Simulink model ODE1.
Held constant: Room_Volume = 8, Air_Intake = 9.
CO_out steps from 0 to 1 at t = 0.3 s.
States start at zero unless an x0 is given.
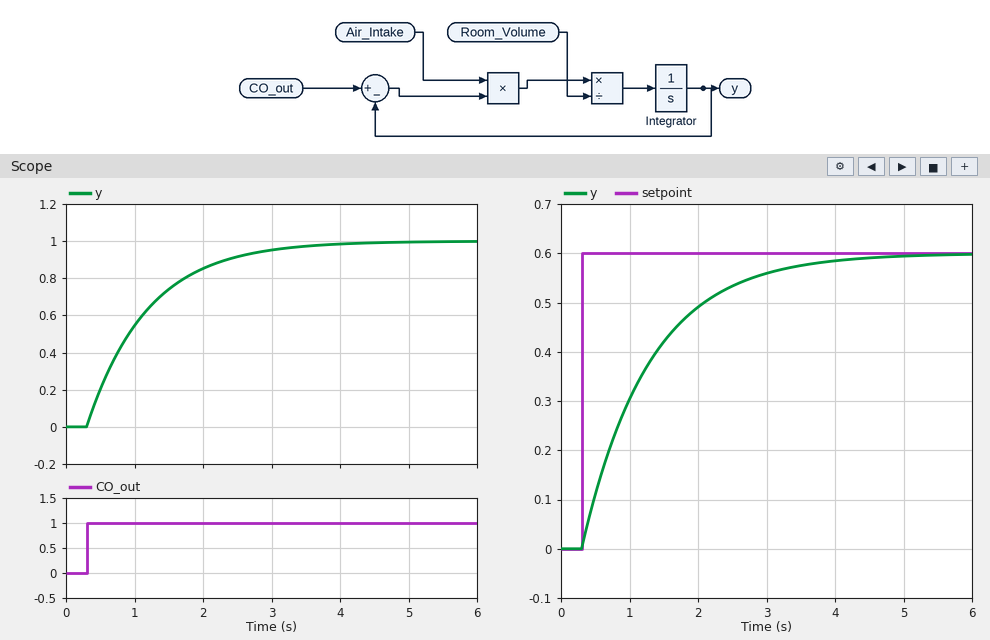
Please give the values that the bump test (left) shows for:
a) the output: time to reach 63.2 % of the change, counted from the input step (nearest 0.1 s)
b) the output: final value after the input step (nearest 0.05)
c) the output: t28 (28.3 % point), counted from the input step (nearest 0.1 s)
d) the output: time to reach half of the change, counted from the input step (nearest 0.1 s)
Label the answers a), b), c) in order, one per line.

a) 0.9 s
b) 1.00
c) 0.3 s
d) 0.6 s
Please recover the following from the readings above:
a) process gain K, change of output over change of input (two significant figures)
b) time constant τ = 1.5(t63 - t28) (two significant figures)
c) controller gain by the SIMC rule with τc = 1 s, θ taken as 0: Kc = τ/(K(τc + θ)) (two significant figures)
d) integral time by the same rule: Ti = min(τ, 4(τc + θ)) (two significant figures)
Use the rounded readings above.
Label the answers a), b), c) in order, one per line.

a) 1.0
b) 0.90 s
c) 0.90
d) 0.90 s
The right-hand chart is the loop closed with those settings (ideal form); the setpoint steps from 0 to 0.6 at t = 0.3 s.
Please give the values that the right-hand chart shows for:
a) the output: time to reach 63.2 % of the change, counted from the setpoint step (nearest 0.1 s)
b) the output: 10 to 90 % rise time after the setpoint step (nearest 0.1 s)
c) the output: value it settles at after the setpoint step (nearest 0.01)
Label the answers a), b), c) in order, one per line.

a) 1.0 s
b) 2.2 s
c) 0.60
